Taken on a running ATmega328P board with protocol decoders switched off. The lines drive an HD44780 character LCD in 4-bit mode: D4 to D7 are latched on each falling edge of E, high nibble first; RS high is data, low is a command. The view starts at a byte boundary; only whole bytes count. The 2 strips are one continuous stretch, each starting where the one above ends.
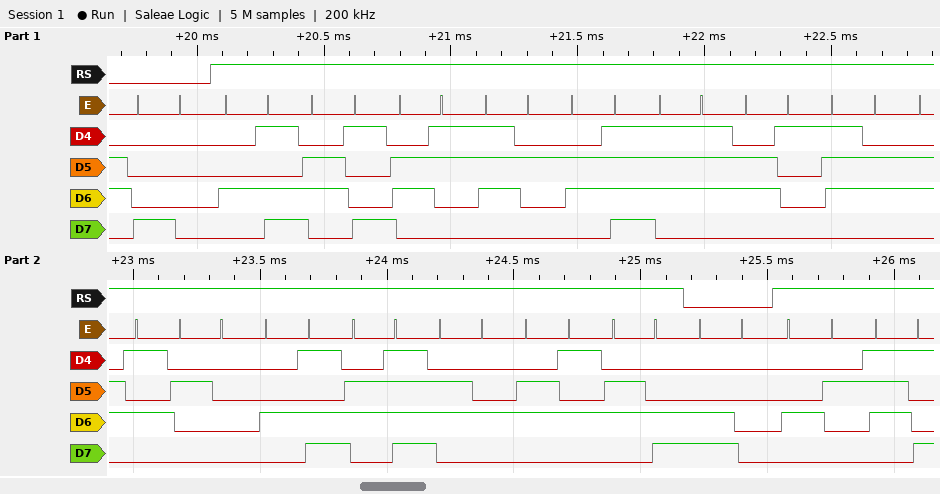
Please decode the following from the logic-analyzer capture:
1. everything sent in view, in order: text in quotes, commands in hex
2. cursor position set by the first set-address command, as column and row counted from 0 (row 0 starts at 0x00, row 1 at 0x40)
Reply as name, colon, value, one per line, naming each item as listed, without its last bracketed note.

everything sent in view, in order: text in quotes, commands in hex: 0x80 "Microwave Model" 0xC0 "By"
cursor position set by the first set-address command, as column and row counted from 0: column 0, row 0
